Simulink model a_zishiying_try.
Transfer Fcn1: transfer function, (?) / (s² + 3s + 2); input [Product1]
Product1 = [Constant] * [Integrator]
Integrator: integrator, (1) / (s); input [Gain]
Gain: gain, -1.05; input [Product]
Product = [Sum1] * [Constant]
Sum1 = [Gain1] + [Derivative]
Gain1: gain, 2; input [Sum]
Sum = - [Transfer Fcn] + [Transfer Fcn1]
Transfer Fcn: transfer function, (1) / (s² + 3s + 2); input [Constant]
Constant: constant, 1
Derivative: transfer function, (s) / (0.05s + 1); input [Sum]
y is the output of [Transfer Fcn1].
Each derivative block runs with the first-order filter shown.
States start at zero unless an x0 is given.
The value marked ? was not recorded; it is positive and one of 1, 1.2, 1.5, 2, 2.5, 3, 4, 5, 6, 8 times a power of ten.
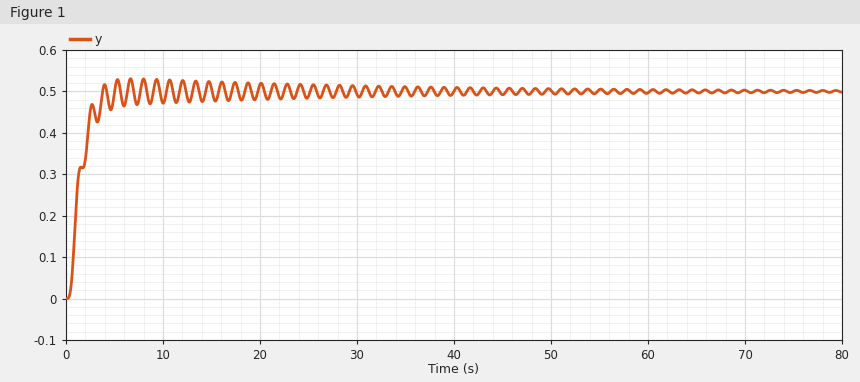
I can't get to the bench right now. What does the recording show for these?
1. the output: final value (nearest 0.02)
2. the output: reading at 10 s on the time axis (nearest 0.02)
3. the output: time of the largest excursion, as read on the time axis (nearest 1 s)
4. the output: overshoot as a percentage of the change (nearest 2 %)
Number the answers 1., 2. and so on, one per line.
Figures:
1. 0.50
2. 0.48
3. 7 s
4. 6 %
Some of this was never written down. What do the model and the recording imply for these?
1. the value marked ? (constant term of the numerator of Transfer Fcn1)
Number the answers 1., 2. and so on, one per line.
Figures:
1. 20
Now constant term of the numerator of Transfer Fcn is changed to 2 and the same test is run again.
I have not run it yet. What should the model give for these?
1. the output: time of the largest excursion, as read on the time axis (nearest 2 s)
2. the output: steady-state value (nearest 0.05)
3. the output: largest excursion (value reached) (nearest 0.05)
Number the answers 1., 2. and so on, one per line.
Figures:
1. 6 s
2. 1.00
3. 1.05
